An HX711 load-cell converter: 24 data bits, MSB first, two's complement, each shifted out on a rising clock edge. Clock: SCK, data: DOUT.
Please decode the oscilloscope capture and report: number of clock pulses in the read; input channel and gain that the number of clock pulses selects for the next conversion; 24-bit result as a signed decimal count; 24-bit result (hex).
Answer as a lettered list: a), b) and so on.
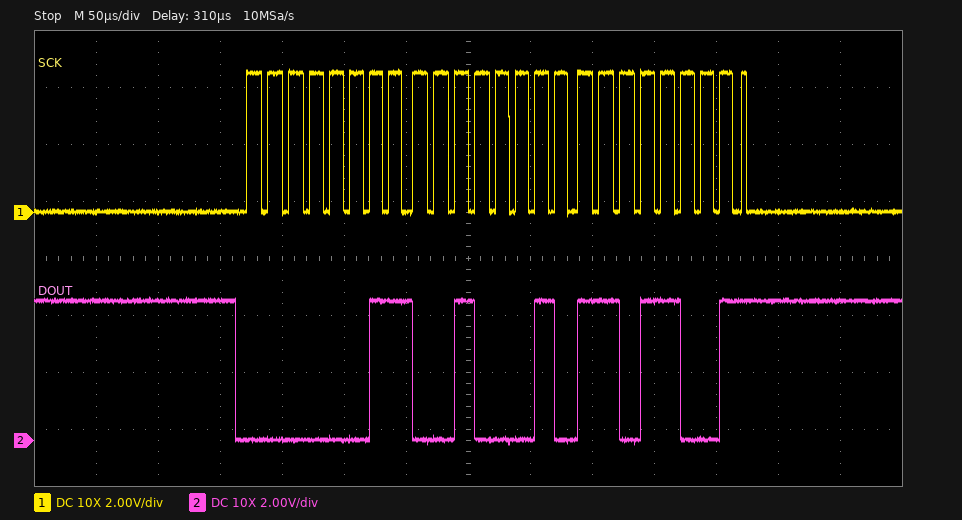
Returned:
a) 25
b) channel A, gain 128
c) 205529
d) 0x0322D9
